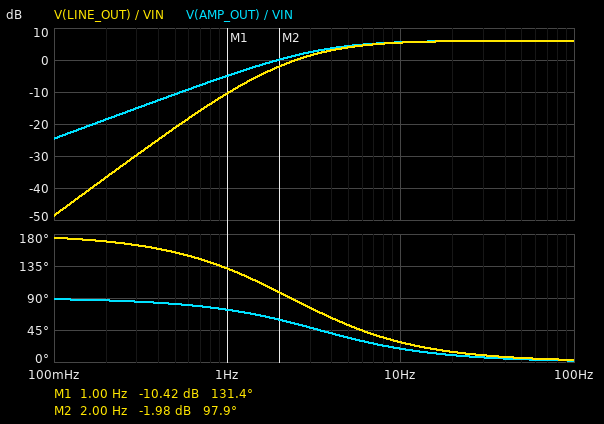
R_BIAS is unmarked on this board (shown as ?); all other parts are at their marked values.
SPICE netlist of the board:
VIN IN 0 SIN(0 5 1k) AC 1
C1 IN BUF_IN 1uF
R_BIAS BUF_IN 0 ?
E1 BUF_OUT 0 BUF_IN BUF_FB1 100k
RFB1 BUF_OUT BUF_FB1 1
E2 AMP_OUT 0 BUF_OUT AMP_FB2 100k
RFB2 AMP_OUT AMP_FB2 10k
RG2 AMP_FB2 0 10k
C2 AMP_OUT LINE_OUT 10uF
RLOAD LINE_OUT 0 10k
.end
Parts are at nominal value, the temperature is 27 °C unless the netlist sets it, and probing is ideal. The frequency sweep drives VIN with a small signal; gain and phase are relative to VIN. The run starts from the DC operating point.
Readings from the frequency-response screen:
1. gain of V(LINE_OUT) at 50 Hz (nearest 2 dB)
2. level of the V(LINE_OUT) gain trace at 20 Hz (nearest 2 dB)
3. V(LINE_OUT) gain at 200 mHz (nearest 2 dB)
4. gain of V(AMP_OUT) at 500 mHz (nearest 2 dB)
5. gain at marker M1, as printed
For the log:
6 dB
6 dB
-36 dB
-10 dB
-10.42 dB
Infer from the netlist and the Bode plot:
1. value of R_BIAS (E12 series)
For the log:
47 kΩ
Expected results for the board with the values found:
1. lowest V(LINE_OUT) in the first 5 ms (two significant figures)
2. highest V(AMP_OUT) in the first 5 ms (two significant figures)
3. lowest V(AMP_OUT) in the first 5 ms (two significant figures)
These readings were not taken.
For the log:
-10 V
10 V
-10 V
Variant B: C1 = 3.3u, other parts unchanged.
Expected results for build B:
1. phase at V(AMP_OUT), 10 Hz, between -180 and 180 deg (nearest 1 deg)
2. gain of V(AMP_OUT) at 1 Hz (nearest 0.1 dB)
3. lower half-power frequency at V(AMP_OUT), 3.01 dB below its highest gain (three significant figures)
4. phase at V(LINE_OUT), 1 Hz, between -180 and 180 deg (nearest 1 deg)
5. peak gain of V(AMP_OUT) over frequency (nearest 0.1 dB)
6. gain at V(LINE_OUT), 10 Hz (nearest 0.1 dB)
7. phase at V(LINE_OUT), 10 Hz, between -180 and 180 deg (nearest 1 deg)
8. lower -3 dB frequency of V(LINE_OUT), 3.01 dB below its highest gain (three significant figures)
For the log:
6 deg
2.9 dB
1.03 Hz
104 deg
6.0 dB
5.9 dB
15 deg
2.05 Hz
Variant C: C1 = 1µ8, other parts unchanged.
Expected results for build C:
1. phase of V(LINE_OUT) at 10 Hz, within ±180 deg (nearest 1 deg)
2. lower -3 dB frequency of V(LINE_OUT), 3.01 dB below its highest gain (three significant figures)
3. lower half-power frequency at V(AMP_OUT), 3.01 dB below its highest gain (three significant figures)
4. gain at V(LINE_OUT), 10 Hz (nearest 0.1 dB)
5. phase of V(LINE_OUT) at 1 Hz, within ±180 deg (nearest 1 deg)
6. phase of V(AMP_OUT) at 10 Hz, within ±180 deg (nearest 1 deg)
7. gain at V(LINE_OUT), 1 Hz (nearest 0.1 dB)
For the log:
20 deg
2.70 Hz
1.88 Hz
5.8 dB
120 deg
11 deg
-6.0 dB
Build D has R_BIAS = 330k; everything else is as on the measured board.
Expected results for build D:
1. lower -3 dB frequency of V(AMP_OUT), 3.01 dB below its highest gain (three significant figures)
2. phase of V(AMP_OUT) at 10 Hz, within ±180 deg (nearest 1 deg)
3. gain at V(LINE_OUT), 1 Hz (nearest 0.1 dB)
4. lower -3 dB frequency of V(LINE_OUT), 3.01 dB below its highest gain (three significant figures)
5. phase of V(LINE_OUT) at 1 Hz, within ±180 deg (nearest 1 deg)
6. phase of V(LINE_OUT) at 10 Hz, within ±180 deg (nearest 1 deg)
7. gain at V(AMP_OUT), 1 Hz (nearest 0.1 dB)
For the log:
482 mHz
3 deg
-0.4 dB
1.72 Hz
84 deg
12 deg
5.1 dB
